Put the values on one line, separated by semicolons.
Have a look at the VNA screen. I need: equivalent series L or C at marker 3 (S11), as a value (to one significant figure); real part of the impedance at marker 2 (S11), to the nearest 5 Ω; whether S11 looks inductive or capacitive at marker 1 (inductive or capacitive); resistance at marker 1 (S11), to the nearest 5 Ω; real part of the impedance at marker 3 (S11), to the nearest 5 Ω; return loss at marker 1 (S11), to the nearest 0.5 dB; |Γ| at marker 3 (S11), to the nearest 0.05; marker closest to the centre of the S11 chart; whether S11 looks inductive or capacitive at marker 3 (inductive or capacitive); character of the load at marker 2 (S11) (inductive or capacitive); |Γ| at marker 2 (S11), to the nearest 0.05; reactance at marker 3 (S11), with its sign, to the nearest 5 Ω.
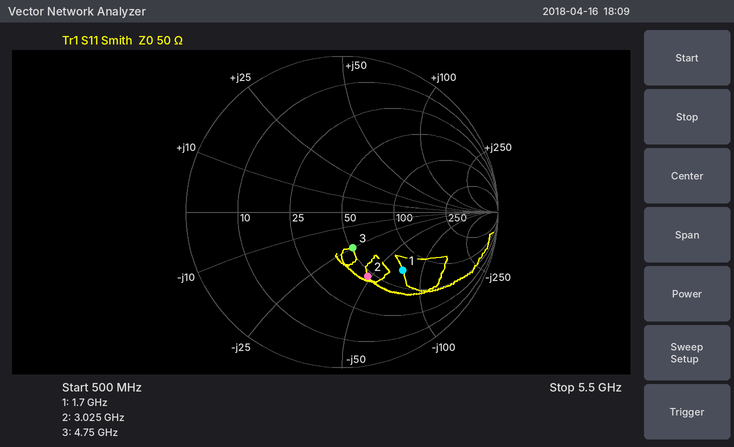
1 pF; 45 Ω; capacitive; 70 Ω; 50 Ω; 5.5 dB; 0.25; marker 3; capacitive; capacitive; 0.45; -25 Ω
